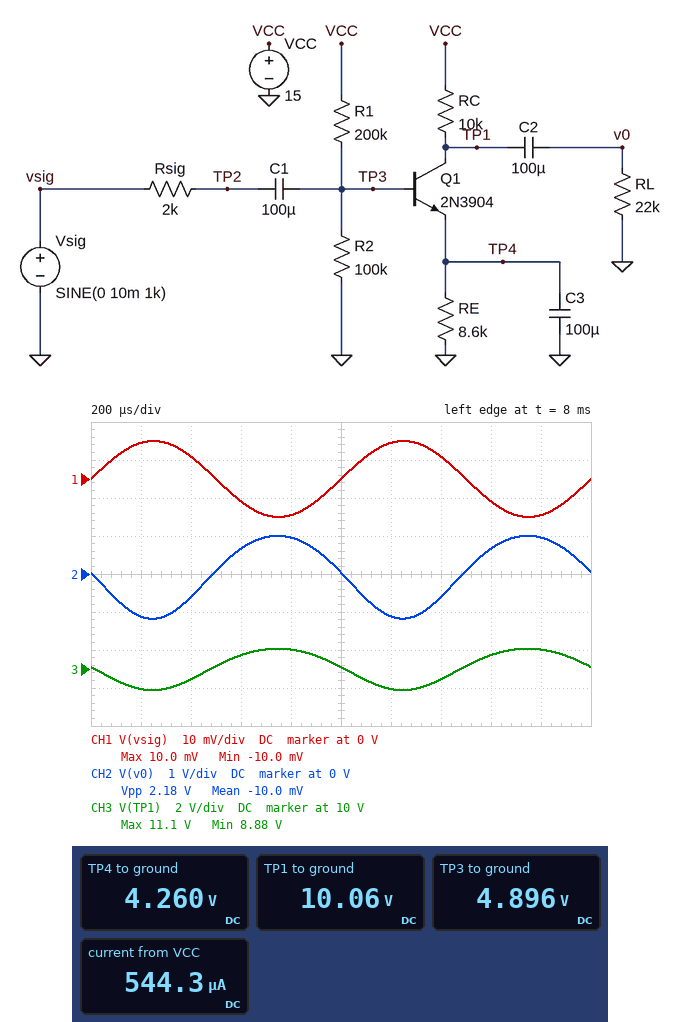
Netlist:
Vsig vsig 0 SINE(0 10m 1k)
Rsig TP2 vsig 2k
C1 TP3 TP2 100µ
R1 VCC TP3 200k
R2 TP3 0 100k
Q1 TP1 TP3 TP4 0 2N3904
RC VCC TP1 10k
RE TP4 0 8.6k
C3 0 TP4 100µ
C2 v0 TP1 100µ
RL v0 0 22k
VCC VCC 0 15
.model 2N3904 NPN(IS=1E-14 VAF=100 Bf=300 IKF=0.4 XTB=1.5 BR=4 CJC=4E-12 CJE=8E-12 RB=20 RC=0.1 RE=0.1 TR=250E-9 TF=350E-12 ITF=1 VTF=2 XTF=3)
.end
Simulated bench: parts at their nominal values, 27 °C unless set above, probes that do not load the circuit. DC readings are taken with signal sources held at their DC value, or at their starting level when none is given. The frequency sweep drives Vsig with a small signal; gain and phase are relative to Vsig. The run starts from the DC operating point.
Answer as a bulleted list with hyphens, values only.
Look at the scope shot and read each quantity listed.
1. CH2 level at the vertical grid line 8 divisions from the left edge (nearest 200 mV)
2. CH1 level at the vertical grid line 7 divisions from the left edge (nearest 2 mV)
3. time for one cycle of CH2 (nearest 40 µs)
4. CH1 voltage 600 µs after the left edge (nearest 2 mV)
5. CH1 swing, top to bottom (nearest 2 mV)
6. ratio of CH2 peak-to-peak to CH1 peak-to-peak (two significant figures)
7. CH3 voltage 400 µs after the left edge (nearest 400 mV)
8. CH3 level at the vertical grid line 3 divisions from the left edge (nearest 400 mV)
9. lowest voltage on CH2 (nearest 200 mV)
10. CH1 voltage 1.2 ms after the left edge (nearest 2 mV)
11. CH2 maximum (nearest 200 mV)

- 600 mV
- 6 mV
- 1.00 ms
- -6 mV
- 20 mV
- 110
- 9.6 V
- 10.8 V
- -1.2 V
- 10 mV
- 1.0 V
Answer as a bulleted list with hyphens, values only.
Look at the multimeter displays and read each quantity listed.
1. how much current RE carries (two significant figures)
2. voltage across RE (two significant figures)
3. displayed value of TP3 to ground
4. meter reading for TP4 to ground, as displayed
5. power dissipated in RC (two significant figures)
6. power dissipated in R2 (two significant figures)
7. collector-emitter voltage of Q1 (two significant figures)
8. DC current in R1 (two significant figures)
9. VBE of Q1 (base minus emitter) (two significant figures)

- 500 µA
- 4.3 V
- 4.896 V
- 4.260 V
- 2.4 mW
- 240 µW
- 5.8 V
- 51 µA
- 640 mV
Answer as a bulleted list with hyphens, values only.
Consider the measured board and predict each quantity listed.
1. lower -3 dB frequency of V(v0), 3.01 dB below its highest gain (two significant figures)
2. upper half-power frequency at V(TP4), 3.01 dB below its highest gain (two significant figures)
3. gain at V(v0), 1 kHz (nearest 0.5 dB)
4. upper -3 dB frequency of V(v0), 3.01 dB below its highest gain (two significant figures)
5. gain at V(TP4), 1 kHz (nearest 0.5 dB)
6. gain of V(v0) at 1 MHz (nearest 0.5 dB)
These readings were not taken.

- 27 Hz
- 27 Hz
- 41.0 dB
- 320 kHz
- -32.0 dB
- 30.5 dB
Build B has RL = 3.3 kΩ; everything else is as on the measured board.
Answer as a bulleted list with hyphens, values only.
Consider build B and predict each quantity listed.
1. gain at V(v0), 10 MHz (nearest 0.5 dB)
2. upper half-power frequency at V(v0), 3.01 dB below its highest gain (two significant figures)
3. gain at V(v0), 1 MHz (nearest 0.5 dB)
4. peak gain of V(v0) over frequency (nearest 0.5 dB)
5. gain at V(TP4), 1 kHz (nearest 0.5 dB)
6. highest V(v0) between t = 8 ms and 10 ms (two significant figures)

- 10.0 dB
- 770 kHz
- 28.0 dB
- 32.0 dB
- -31.5 dB
- 370 mV
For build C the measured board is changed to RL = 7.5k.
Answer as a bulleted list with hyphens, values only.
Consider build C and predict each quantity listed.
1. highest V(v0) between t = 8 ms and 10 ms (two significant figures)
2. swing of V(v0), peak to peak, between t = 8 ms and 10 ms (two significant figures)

- 630 mV
- 1.4 V
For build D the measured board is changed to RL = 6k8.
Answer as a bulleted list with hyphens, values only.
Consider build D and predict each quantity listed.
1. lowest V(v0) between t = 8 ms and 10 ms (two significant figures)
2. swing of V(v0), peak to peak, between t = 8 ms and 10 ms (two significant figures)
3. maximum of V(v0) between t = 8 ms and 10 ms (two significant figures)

- -700 mV
- 1.3 V
- 600 mV
